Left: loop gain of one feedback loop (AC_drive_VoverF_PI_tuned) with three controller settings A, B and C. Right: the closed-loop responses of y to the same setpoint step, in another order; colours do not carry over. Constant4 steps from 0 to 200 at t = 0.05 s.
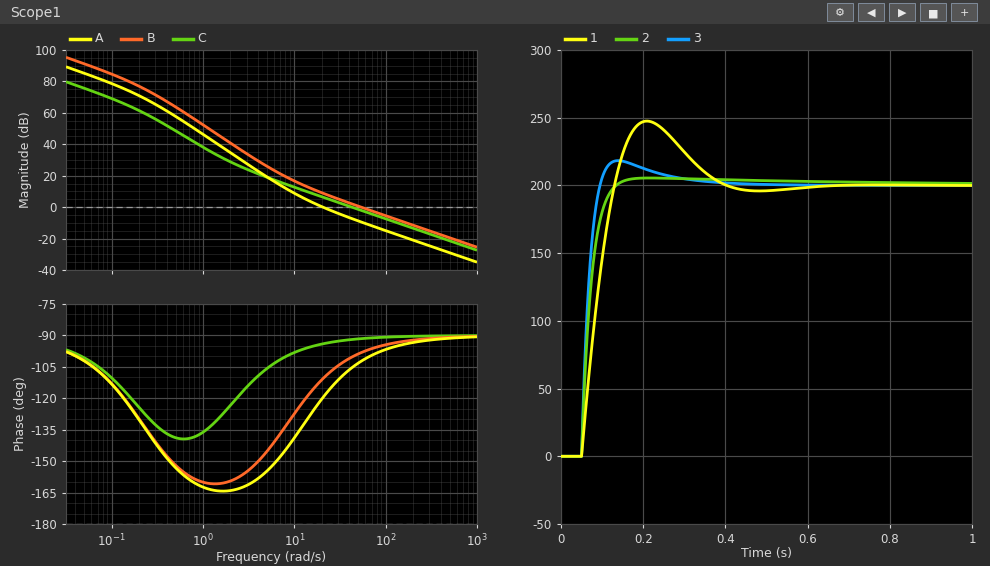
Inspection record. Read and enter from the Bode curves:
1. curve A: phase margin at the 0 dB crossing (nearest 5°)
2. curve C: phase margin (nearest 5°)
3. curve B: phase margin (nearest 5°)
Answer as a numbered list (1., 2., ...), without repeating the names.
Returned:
1. 60°
2. 90°
3. 80°
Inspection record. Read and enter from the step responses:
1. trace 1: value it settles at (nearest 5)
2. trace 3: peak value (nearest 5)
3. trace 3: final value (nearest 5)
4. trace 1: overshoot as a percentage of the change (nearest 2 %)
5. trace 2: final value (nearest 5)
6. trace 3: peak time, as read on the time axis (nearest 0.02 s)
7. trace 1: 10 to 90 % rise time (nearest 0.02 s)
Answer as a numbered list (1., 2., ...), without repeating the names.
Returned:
1. 200
2. 220
3. 200
4. 24 %
5. 200
6. 0.14 s
7. 0.06 s
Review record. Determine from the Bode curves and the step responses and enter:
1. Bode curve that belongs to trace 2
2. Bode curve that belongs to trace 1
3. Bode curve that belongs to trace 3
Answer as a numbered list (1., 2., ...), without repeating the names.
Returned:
1. C
2. A
3. B
